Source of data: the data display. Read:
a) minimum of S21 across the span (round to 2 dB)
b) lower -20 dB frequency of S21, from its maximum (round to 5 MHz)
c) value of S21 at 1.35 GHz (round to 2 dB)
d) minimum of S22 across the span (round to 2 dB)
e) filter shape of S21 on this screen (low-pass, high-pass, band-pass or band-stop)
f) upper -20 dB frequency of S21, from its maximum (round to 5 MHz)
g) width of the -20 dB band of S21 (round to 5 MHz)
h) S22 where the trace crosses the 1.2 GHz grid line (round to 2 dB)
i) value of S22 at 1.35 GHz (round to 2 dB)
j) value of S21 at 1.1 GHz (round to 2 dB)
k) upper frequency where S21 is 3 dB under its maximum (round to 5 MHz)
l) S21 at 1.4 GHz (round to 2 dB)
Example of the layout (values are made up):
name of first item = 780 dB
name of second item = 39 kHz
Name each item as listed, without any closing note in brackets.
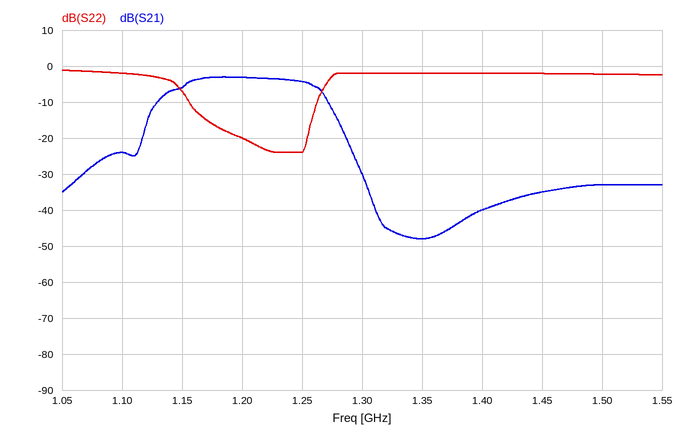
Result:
minimum of S21 across the span = -48 dB
lower -20 dB frequency of S21, from its maximum = 1.115 GHz
value of S21 at 1.35 GHz = -48 dB
minimum of S22 across the span = -24 dB
filter shape of S21 on this screen = band-pass
upper -20 dB frequency of S21, from its maximum = 1.290 GHz
width of the -20 dB band of S21 = 175 MHz
S22 where the trace crosses the 1.2 GHz grid line = -20 dB
value of S22 at 1.35 GHz = -2 dB
value of S21 at 1.1 GHz = -24 dB
upper frequency where S21 is 3 dB under its maximum = 1.265 GHz
S21 at 1.4 GHz = -40 dB
